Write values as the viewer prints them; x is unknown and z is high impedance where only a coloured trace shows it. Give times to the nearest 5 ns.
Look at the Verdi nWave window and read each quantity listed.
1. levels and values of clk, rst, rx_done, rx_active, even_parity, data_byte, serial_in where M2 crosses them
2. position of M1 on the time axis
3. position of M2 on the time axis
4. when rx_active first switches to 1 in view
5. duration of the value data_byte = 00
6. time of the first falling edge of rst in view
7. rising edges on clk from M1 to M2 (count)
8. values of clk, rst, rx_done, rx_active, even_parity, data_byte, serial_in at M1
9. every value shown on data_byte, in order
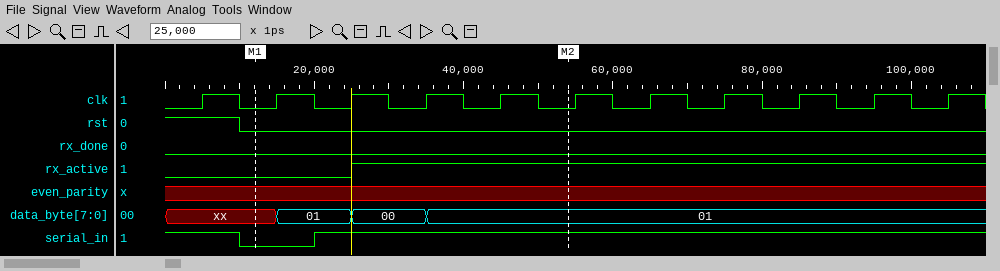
clk=0, rst=0, rx_done=0, rx_active=1, even_parity=x, data_byte=01, serial_in=1
10 ns
55 ns
25 ns
10 ns
10 ns
4
clk=0, rst=0, rx_done=0, rx_active=0, even_parity=x, data_byte=xx, serial_in=0
xx, 01, 00, 01
